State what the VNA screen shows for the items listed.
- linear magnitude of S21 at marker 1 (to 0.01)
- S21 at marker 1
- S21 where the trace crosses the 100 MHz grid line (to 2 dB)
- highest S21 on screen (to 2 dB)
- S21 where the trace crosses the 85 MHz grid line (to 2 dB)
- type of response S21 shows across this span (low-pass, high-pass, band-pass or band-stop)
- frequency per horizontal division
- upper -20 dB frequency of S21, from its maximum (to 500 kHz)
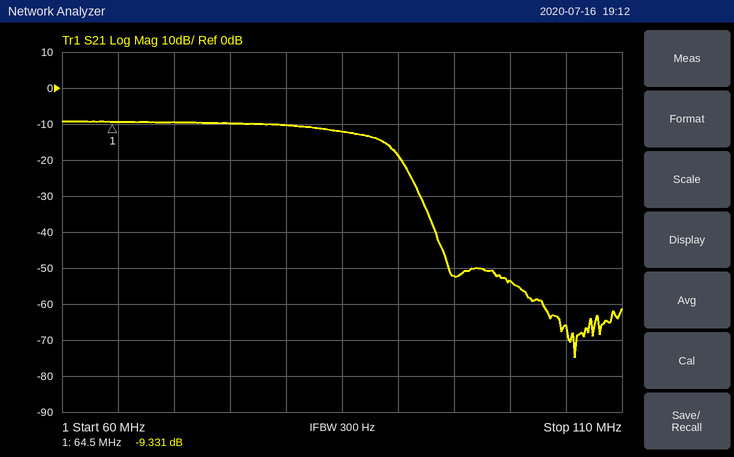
0.34
-9.331 dB
-54 dB
-10 dB
-12 dB
low-pass
5 MHz
92.0 MHz
